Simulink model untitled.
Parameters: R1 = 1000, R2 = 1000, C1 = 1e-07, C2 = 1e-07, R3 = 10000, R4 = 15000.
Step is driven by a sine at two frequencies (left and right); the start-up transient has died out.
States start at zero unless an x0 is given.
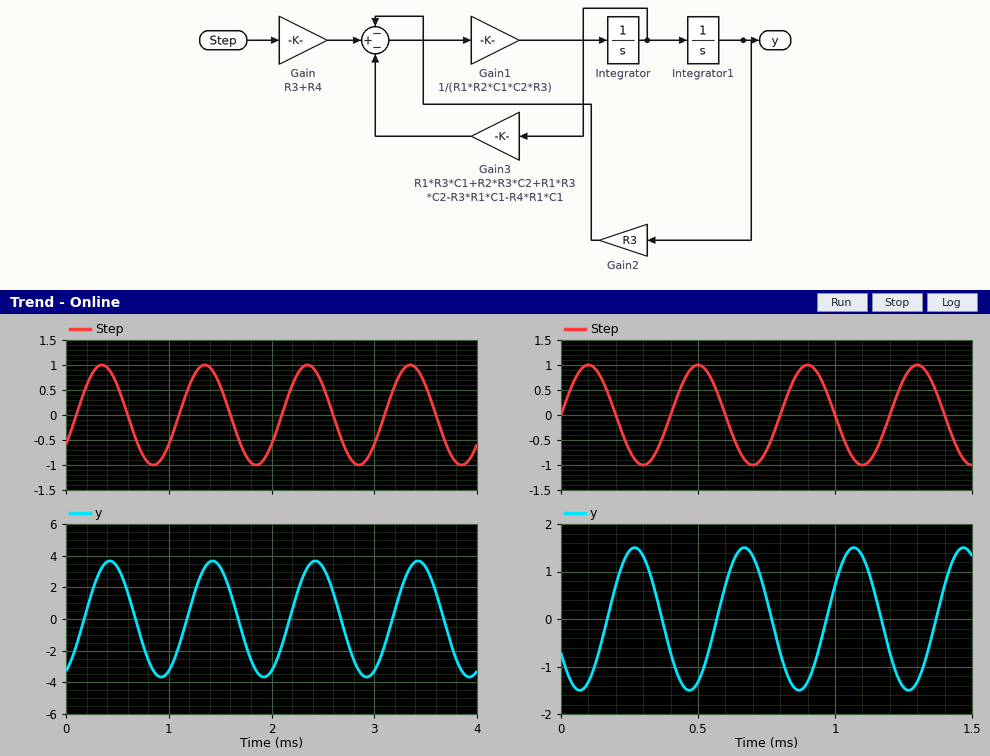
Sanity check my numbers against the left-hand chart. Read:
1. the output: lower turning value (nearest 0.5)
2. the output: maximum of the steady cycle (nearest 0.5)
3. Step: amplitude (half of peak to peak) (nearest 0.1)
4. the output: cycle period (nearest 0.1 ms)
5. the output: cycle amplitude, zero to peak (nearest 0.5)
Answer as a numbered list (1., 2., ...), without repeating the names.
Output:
1. -3.5
2. 3.5
3. 1.0
4. 1.0 ms
5. 3.5
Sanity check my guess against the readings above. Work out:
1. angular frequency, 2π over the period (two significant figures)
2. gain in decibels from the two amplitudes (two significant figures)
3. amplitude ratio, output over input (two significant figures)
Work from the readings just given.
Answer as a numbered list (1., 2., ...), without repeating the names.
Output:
1. 6.3 rad/ms
2. 11 dB
3. 3.5
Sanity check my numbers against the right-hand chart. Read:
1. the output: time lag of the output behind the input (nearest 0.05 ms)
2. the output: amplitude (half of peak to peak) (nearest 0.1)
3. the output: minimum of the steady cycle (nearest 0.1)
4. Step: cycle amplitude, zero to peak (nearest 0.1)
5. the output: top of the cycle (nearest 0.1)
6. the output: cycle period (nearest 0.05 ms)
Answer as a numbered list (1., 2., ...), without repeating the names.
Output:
1. 0.15 ms
2. 1.5
3. -1.5
4. 1.0
5. 1.5
6. 0.40 ms
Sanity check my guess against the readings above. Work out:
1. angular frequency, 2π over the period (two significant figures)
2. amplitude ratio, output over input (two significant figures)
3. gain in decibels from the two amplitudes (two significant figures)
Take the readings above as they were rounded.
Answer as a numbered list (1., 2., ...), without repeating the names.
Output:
1. 16 rad/ms
2. 1.5
3. 3.5 dB
